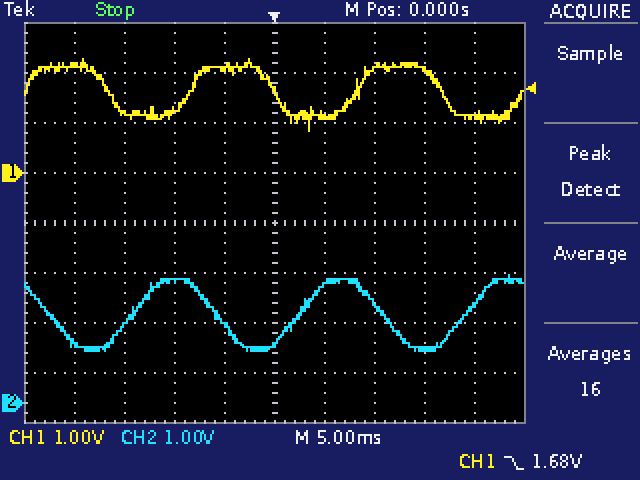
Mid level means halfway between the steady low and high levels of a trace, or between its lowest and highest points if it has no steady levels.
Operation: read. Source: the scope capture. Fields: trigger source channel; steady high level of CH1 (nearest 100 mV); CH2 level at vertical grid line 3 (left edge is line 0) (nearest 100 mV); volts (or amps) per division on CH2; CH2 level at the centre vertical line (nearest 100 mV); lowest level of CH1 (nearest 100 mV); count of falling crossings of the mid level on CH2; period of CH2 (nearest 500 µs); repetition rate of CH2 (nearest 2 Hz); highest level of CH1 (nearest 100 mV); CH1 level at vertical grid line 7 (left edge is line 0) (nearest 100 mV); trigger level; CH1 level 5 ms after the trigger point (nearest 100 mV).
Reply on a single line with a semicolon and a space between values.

CH1; 2.1 V; 2.4 V; 1 V; 1.2 V; 800 mV; 3; 16.5 ms; 60 Hz; 2.3 V; 2.1 V; 1.68 V; 1.2 V
